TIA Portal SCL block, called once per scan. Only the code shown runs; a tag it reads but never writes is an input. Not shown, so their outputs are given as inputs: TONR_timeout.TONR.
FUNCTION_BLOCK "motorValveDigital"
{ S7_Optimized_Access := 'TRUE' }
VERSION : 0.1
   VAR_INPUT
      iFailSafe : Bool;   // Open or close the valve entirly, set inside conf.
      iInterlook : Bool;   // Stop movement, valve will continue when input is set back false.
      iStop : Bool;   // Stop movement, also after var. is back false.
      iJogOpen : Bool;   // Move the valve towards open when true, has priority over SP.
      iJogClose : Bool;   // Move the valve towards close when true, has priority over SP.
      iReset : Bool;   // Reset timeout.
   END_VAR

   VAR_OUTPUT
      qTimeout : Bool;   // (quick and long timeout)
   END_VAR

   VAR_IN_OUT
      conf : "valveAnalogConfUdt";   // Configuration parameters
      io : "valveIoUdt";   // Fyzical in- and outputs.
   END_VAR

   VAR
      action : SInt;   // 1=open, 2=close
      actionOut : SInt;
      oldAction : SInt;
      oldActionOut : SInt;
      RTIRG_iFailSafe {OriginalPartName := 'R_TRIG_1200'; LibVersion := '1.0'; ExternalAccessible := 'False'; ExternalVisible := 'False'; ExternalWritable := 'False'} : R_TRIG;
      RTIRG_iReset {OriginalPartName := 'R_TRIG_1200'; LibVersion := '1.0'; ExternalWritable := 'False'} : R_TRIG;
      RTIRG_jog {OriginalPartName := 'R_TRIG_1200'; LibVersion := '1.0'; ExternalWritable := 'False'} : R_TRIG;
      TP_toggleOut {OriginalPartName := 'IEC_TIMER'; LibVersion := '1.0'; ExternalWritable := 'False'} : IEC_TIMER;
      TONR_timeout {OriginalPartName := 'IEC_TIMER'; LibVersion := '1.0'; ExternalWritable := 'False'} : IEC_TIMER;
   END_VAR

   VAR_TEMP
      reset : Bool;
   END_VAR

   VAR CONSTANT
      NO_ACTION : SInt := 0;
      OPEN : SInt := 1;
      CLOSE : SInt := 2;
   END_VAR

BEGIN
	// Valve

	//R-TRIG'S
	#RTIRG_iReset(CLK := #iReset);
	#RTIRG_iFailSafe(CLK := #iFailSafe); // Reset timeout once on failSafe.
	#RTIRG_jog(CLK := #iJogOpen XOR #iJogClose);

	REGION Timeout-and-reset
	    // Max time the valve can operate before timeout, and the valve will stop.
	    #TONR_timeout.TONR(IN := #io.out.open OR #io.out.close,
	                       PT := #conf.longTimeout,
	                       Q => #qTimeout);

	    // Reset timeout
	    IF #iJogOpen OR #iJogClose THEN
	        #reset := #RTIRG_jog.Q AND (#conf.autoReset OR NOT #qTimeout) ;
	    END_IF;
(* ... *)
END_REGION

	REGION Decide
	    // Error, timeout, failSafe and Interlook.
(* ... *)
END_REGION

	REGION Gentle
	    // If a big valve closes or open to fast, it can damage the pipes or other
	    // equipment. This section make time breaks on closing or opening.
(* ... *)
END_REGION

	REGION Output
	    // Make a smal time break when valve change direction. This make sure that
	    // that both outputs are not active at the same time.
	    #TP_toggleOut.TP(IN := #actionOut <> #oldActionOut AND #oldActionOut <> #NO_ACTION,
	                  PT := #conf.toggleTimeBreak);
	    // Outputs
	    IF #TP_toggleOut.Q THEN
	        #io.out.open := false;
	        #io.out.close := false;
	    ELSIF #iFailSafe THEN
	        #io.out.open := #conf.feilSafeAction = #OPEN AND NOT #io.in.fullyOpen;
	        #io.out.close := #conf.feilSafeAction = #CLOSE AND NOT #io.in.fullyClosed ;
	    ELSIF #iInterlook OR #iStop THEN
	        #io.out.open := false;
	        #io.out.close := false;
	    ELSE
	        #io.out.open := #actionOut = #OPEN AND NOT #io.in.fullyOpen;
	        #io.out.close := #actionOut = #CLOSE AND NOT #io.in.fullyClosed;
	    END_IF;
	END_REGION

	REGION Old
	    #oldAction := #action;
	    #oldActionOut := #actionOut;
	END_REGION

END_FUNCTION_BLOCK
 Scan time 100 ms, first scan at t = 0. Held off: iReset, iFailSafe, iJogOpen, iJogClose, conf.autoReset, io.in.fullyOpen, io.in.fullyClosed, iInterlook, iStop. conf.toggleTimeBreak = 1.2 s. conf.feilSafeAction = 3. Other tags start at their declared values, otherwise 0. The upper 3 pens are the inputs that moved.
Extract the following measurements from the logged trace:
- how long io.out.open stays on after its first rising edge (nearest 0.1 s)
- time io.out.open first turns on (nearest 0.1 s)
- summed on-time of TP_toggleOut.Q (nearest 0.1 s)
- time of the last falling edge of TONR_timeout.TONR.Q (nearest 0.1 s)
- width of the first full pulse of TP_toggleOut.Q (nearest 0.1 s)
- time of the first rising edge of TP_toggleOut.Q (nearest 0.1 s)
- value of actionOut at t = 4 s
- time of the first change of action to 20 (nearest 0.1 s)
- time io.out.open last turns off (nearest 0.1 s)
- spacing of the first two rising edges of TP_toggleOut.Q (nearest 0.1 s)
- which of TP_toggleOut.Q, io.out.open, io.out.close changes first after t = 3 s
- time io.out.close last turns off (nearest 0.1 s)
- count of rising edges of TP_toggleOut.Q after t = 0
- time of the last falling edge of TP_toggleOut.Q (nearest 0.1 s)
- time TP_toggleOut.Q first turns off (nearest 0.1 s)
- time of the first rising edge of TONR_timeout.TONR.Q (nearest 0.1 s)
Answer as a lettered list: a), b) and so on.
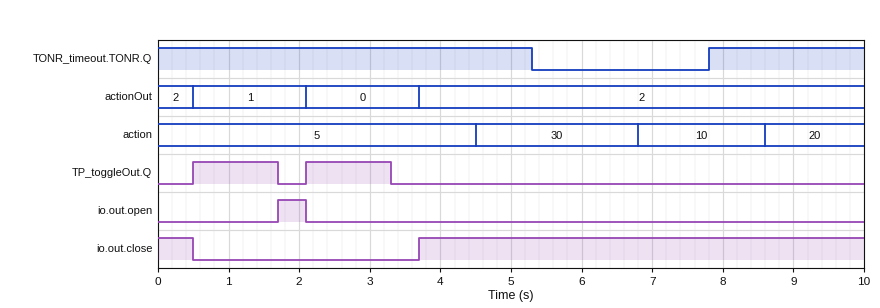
a) 0.4 s
b) 1.7 s
c) 2.4 s
d) 5.3 s
e) 1.2 s
f) 0.5 s
g) 2
h) 8.6 s
i) 2.1 s
j) 1.6 s
k) TP_toggleOut.Q
l) 0.5 s
m) 2
n) 3.3 s
o) 1.7 s
p) 7.8 s
